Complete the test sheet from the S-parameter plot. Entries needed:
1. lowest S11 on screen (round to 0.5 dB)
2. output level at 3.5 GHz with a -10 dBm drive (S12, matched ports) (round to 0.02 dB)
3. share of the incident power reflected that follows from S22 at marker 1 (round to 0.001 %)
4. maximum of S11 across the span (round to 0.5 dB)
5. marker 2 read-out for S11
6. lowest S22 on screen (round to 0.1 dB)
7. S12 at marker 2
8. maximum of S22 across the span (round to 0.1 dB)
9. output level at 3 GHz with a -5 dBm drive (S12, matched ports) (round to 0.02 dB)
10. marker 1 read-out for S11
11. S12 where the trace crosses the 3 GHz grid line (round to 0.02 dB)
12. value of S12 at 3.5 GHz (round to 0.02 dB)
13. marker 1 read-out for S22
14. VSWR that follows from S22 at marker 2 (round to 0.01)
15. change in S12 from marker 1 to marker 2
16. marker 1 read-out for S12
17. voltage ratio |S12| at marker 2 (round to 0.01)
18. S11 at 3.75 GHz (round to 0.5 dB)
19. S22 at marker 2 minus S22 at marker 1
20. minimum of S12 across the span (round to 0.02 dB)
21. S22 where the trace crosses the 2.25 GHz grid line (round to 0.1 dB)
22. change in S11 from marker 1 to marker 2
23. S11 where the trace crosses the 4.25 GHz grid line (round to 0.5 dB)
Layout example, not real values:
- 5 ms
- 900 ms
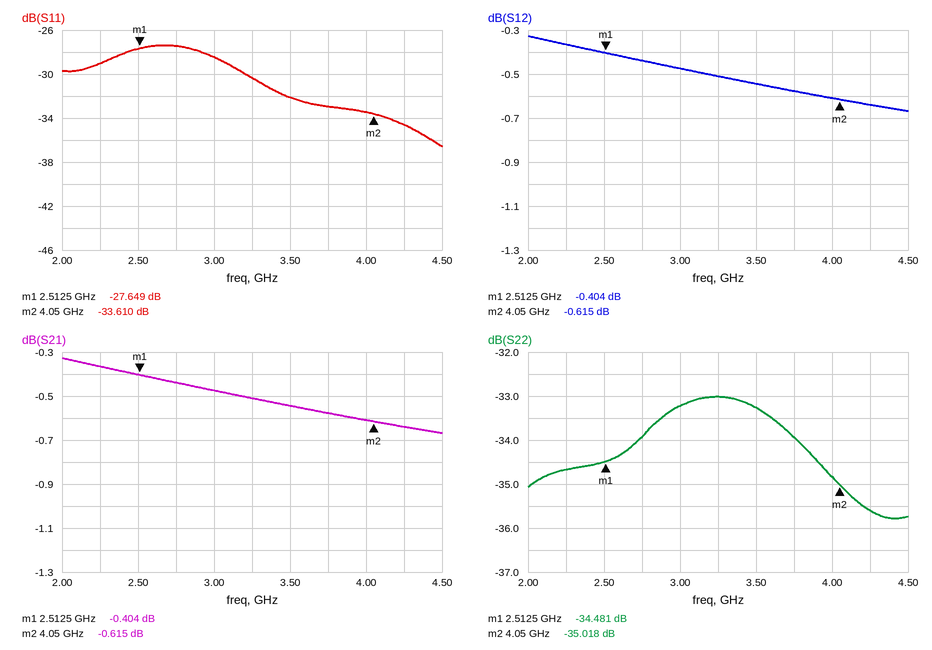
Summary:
- -36.5 dB
- -10.54 dBm
- 0.036 %
- -27.5 dB
- -33.610 dB
- -35.8 dB
- -0.615 dB
- -33.0 dB
- -5.48 dBm
- -27.649 dB
- -0.48 dB
- -0.54 dB
- -34.481 dB
- 1.04
- -0.211 dB
- -0.404 dB
- 0.93
- -33.0 dB
- -0.537 dB
- -0.66 dB
- -34.7 dB
- -5.961 dB
- -34.5 dB
